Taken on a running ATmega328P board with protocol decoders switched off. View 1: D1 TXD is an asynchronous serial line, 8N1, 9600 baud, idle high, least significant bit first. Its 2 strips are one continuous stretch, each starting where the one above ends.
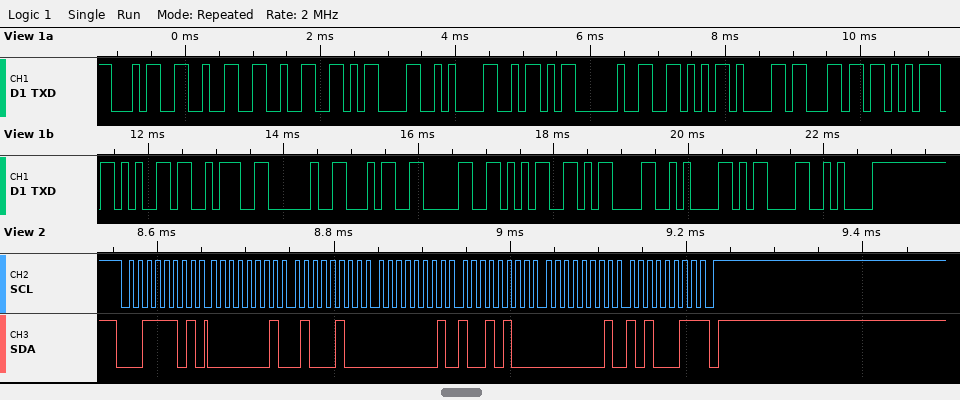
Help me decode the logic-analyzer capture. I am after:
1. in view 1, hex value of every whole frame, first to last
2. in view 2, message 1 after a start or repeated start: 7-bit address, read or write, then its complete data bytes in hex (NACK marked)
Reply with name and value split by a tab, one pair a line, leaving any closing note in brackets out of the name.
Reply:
in view 1, hex value of every whole frame, first to last	34 32 32 0D 0A 5A 20 56 61 6C 75 65 3A 20 34 30 35 0D 0A 0D 0A
in view 2, message 1 after a start or repeated start: 7-bit address, read or write, then its complete data bytes in hex	0x1E read: 01 44 01 94 01 A3 NACK
